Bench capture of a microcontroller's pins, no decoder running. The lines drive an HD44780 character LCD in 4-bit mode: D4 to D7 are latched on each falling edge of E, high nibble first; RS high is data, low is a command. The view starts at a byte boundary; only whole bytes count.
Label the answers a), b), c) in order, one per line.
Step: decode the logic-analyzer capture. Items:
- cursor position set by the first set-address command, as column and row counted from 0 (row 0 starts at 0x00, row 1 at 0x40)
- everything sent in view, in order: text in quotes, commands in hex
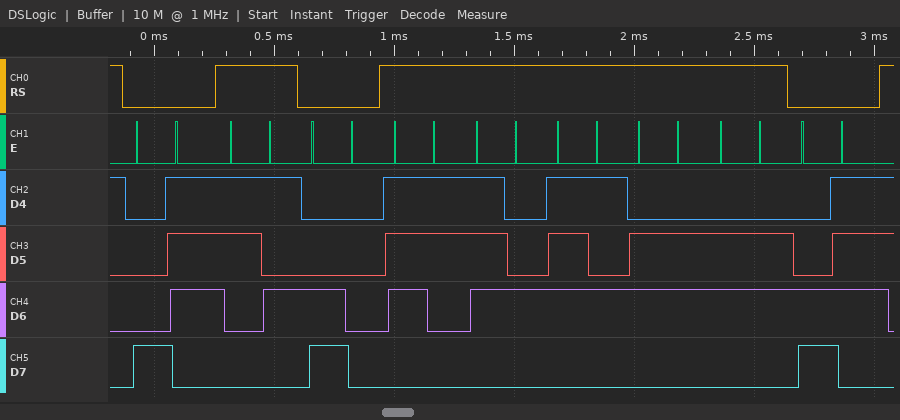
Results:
a) column 7, row 0
b) 0x87 "5" 0xC0 "stuff" 0xC7
